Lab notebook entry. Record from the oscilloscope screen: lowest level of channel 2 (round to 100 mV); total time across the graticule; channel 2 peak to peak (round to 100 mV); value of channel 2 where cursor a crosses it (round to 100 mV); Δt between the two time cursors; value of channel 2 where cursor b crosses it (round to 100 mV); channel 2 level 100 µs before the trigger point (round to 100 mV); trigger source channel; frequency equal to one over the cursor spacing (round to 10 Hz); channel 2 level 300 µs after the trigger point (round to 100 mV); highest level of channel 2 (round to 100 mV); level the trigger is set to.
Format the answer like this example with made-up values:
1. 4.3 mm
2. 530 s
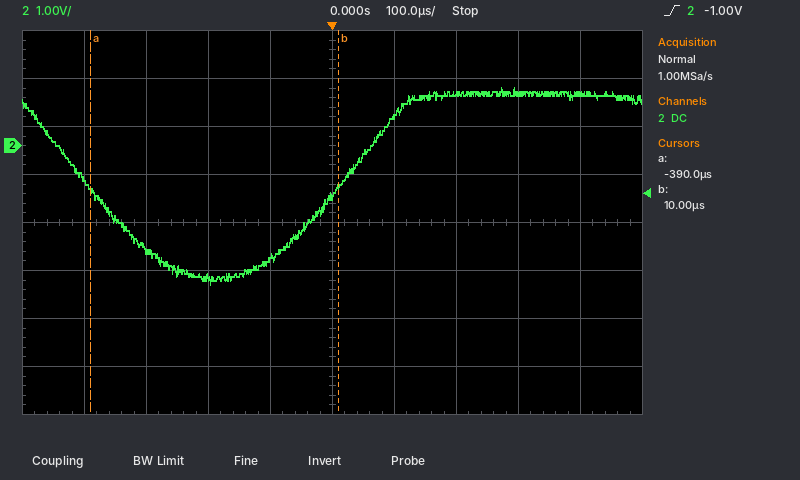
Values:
1. -2.9 V
2. 1 ms
3. 4.1 V
4. -900 mV
5. 400 µs
6. -900 mV
7. -2.3 V
8. channel 2
9. 2.50 kHz
10. 1.1 V
11. 1.2 V
12. -1.00 V
